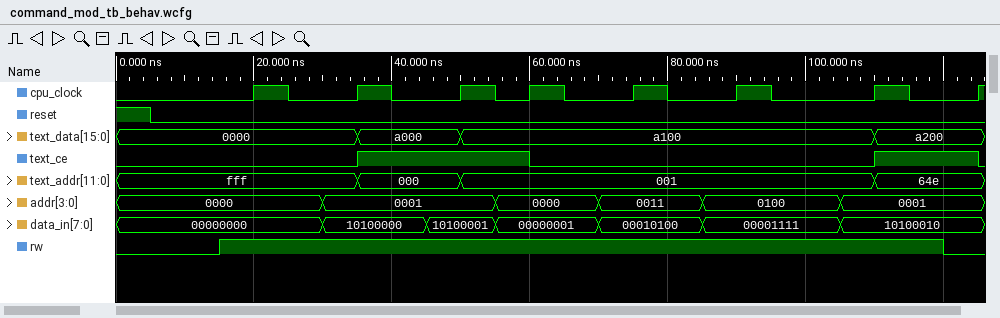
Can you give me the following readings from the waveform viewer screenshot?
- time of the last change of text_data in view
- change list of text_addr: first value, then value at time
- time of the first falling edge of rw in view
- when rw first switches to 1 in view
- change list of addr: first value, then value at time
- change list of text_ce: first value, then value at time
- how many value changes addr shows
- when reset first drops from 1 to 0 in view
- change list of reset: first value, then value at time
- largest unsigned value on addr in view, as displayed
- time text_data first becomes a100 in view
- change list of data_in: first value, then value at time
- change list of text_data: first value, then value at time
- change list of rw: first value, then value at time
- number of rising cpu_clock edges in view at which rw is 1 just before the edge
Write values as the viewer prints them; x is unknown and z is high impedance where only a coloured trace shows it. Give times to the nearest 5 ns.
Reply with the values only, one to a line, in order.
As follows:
110 ns
fff, 000 at 35 ns, 001 at 50 ns, 64e at 110 ns
120 ns
15 ns
0000, 0001 at 30 ns, 0000 at 55 ns, 0011 at 70 ns, 0100 at 85 ns, 0001 at 105 ns
0, 1 at 35 ns, 0 at 60 ns, 1 at 110 ns, 0 at 125 ns
5
5 ns
1, 0 at 5 ns
0100
50 ns
00000000, 10100000 at 30 ns, 10100001 at 45 ns, 00000001 at 55 ns, 00010100 at 70 ns, 00001111 at 85 ns, 10100010 at 105 ns
0000, a000 at 35 ns, a100 at 50 ns, a200 at 110 ns
0, 1 at 15 ns, 0 at 120 ns
7
